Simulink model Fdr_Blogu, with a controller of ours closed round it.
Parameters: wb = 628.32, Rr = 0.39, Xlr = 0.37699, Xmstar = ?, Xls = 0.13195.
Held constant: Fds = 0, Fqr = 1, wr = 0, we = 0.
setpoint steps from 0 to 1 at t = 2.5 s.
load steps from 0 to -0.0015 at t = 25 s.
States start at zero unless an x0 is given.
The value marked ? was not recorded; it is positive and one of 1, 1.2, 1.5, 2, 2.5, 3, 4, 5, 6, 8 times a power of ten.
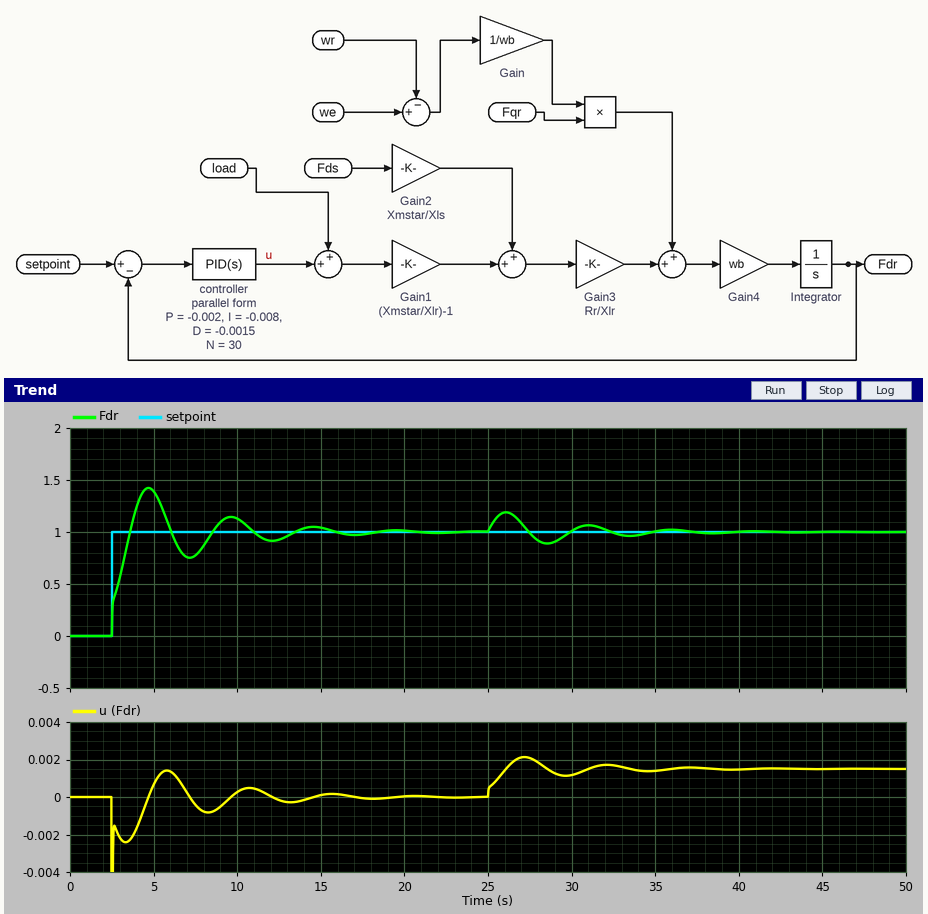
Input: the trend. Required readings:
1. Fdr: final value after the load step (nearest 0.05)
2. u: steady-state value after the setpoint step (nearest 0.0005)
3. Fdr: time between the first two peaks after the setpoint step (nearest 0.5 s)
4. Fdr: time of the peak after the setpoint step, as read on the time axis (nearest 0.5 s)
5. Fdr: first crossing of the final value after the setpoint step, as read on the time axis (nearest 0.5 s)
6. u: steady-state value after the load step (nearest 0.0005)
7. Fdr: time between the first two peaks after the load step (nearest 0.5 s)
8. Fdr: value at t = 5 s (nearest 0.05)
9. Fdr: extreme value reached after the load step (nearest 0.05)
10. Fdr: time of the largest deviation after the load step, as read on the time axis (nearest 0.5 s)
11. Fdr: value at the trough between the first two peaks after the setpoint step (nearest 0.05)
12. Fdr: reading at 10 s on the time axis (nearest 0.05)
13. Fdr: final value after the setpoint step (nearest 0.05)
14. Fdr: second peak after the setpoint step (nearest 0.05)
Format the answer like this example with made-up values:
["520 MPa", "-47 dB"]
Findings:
["1.00", "0.0000", "5.0 s", "4.5 s", "3.5 s", "0.0015", "5.0 s", "1.40", "1.20", "26.0 s", "0.75", "1.15", "1.00", "1.15"]
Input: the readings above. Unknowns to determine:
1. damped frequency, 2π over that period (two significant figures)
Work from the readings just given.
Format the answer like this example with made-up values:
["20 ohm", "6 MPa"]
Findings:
["1.3 rad/s"]
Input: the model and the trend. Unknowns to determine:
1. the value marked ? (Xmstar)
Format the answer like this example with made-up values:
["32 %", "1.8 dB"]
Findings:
["0.2"]
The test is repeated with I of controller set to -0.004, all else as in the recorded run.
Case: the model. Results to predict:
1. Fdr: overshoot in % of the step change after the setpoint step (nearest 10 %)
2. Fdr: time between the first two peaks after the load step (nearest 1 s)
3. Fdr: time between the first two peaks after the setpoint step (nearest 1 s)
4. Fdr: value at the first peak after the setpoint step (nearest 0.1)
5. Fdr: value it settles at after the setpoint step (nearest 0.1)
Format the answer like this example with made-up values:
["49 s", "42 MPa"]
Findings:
["40 %", "7 s", "7 s", "1.4", "1.0"]
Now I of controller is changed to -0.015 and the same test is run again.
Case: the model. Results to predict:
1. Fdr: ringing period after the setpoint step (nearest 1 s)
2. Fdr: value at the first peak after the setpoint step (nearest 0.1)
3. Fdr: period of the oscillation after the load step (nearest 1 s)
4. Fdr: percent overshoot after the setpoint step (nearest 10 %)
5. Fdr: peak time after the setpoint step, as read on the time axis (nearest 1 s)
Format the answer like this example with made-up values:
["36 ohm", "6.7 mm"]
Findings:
["4 s", "1.5", "4 s", "50 %", "4 s"]
